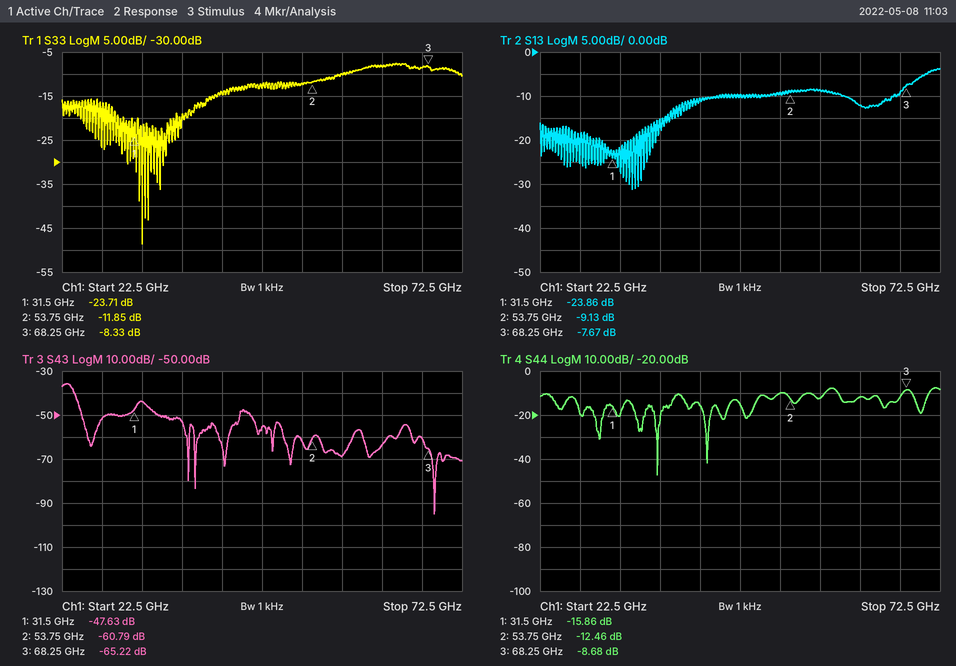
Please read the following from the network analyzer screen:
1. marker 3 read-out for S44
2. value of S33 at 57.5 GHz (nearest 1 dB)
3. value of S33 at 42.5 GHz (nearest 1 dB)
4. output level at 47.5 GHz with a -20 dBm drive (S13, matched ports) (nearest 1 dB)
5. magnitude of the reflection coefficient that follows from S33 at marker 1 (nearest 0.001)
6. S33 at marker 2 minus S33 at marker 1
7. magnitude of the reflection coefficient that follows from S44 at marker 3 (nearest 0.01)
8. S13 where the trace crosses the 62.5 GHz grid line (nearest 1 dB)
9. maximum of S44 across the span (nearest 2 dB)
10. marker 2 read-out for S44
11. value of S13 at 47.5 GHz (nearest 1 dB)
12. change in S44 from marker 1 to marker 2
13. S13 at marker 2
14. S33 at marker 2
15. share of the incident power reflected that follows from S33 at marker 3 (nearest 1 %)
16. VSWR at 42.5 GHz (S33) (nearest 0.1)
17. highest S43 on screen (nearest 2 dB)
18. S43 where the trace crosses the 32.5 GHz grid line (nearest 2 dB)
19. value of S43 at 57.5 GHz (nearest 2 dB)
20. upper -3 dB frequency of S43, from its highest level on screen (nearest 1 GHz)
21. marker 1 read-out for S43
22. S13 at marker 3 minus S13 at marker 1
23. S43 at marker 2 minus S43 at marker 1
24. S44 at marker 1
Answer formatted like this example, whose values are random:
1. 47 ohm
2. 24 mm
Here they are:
1. -8.68 dB
2. -10 dB
3. -14 dB
4. -30 dBm
5. 0.065
6. 11.86 dB
7. 0.37
8. -12 dB
9. -8 dB
10. -12.46 dB
11. -10 dB
12. 3.40 dB
13. -9.13 dB
14. -11.85 dB
15. 15 %
16. 1.5
17. -36 dB
18. -44 dB
19. -68 dB
20. 24 GHz
21. -47.63 dB
22. 16.19 dB
23. -13.16 dB
24. -15.86 dB
